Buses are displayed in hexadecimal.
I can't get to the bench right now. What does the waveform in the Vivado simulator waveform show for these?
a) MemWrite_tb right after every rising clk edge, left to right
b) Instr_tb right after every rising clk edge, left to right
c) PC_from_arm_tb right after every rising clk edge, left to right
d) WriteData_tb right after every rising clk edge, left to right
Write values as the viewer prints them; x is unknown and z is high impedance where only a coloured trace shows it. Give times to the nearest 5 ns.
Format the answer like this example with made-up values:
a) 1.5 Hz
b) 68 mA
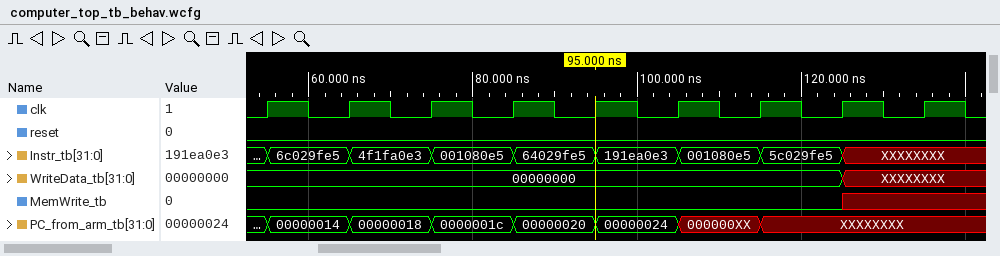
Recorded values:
a) 0 0 0 0 0 0 0 x x
b) 6c029fe5, 4f1fa0e3, 001080e5, 64029fe5, 191ea0e3, 001080e5, 5c029fe5, XXXXXXXX, XXXXXXXX
c) 00000014, 00000018, 0000001c, 00000020, 00000024, 000000XX, XXXXXXXX, XXXXXXXX, XXXXXXXX
d) 00000000, 00000000, 00000000, 00000000, 00000000, 00000000, 00000000, XXXXXXXX, XXXXXXXX
